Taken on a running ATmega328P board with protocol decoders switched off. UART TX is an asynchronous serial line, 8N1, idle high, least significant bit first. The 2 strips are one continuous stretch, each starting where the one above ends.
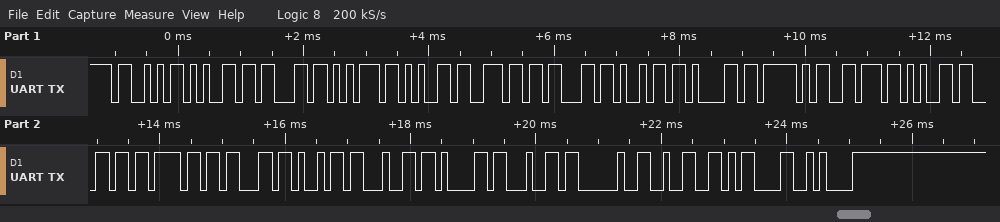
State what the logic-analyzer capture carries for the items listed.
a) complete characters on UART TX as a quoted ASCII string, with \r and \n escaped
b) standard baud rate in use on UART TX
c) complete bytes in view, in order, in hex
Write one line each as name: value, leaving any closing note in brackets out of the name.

complete characters on UART TX as a quoted ASCII string, with \r and \n escaped: "Secuencia_velocidad 2\r\n"
standard baud rate in use on UART TX: 9600 baud
complete bytes in view, in order, in hex: 53 65 63 75 65 6E 63 69 61 5F 76 65 6C 6F 63 69 64 61 64 20 32 0D 0A
